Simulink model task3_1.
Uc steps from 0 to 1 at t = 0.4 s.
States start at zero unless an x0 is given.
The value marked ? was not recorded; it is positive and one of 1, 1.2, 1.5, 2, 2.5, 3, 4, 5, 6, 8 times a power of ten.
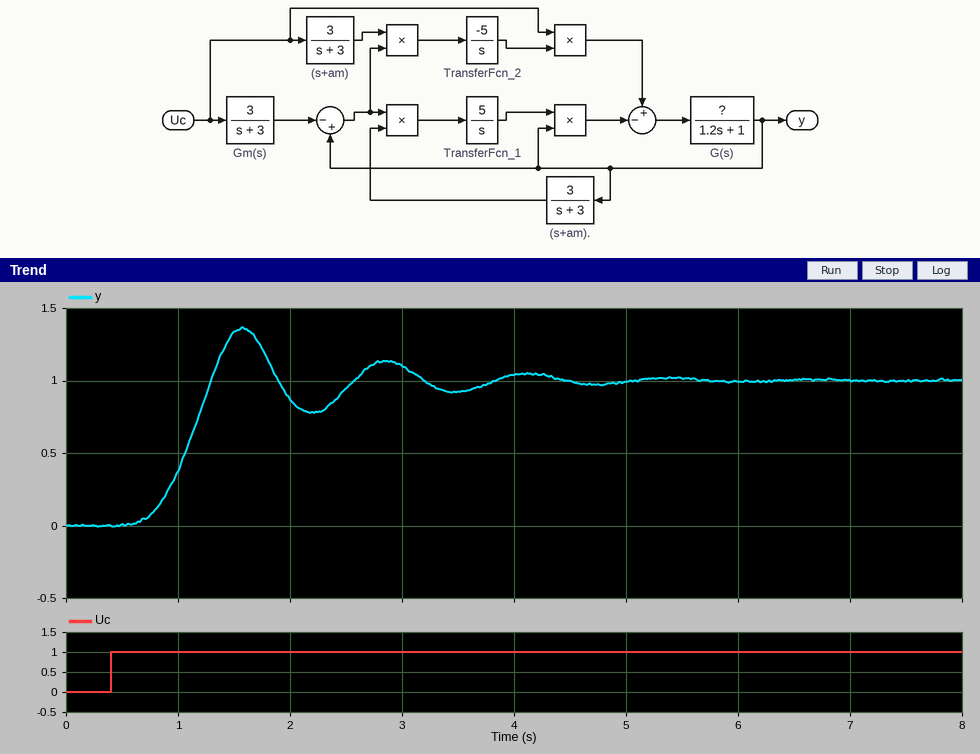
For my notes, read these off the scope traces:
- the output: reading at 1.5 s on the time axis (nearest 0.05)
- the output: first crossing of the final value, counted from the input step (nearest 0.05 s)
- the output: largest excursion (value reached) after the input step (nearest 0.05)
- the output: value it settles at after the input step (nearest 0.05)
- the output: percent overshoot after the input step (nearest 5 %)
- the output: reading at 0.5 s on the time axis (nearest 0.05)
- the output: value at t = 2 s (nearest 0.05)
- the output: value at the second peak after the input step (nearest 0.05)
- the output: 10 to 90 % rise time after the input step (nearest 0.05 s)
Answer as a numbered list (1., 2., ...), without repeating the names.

1. 1.35
2. 0.90 s
3. 1.35
4. 1.00
5. 35 %
6. 0.00
7. 0.85
8. 1.15
9. 0.45 s
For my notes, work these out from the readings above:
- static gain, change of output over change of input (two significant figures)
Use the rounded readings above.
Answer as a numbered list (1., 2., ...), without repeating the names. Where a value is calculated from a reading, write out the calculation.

1. (1 - 0) / (1 - 0) = 1.0
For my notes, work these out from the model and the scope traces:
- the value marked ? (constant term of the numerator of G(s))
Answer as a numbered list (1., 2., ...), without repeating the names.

1. 3
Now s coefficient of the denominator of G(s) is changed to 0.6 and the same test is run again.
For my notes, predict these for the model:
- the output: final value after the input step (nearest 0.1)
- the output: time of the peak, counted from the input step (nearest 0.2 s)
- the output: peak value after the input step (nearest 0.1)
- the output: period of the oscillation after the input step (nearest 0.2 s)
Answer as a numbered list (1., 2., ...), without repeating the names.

1. 1.0
2. 1.0 s
3. 1.2
4. 1.0 s
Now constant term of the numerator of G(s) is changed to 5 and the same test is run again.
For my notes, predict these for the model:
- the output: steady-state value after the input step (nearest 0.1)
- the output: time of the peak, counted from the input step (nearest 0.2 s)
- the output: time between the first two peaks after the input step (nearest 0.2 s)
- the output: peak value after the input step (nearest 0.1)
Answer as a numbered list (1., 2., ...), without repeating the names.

1. 1.0
2. 1.0 s
3. 1.0 s
4. 1.3
